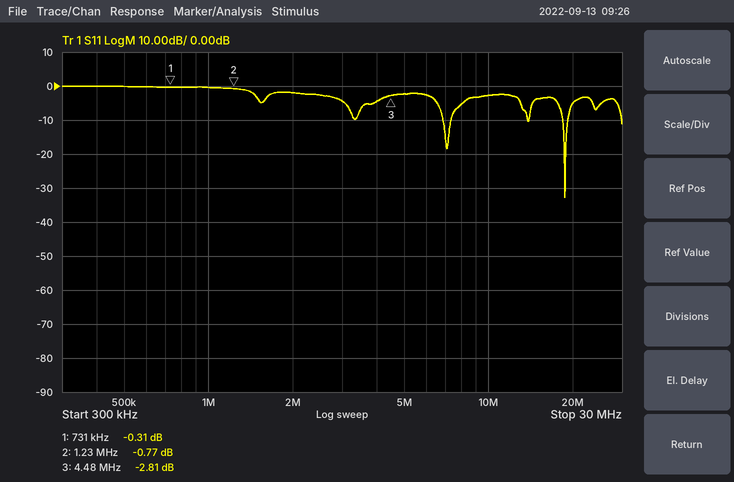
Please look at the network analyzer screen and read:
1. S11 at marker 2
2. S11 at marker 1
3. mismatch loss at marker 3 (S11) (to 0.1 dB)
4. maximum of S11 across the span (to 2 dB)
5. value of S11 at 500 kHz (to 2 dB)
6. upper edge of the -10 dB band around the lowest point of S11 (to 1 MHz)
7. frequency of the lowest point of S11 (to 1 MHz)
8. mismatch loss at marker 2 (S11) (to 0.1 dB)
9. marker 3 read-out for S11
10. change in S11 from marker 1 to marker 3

-0.77 dB
-0.31 dB
3.2 dB
0 dB
0 dB
19 MHz
19 MHz
7.9 dB
-2.81 dB
-2.50 dB
